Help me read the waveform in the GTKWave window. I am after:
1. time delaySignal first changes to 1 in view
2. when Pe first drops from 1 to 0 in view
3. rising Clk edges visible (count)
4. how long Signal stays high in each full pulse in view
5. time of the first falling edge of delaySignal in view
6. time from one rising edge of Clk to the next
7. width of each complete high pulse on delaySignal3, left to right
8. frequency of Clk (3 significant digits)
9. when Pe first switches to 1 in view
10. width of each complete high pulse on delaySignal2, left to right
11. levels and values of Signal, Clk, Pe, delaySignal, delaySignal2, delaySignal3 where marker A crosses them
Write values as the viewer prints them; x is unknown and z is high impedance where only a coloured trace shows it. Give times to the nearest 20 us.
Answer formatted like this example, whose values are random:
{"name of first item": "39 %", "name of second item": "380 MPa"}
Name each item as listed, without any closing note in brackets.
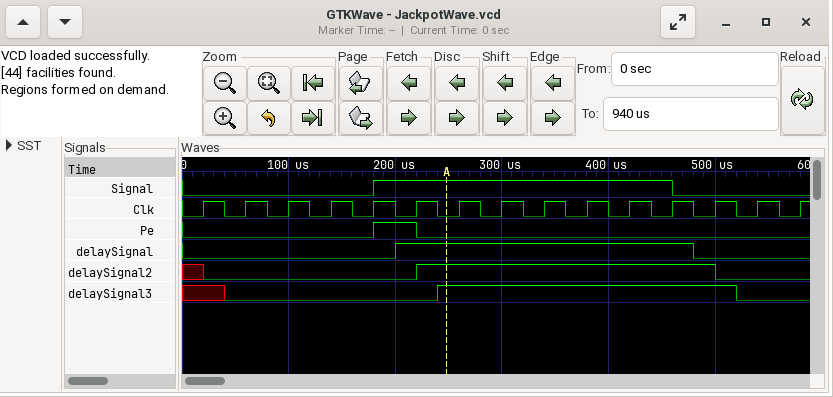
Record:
{"time delaySignal first changes to 1 in view": "200 us", "when Pe first drops from 1 to 0 in view": "220 us", "rising Clk edges visible": "15", "how long Signal stays high in each full pulse in view": "280 us", "time of the first falling edge of delaySignal in view": "480 us", "time from one rising edge of Clk to the next": "40 us", "width of each complete high pulse on delaySignal3, left to right": "280 us", "frequency of Clk": "25.0 kHz", "when Pe first switches to 1 in view": "180 us", "width of each complete high pulse on delaySignal2, left to right": "280 us", "levels and values of Signal, Clk, Pe, delaySignal, delaySignal2, delaySignal3 where marker A crosses them": "Signal=1, Clk=0, Pe=0, delaySignal=1, delaySignal2=1, delaySignal3=1"}
